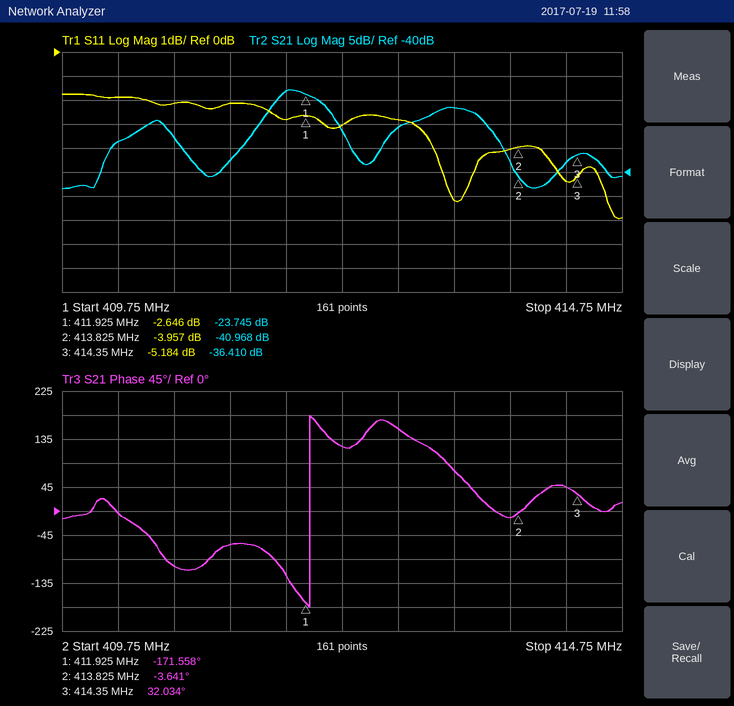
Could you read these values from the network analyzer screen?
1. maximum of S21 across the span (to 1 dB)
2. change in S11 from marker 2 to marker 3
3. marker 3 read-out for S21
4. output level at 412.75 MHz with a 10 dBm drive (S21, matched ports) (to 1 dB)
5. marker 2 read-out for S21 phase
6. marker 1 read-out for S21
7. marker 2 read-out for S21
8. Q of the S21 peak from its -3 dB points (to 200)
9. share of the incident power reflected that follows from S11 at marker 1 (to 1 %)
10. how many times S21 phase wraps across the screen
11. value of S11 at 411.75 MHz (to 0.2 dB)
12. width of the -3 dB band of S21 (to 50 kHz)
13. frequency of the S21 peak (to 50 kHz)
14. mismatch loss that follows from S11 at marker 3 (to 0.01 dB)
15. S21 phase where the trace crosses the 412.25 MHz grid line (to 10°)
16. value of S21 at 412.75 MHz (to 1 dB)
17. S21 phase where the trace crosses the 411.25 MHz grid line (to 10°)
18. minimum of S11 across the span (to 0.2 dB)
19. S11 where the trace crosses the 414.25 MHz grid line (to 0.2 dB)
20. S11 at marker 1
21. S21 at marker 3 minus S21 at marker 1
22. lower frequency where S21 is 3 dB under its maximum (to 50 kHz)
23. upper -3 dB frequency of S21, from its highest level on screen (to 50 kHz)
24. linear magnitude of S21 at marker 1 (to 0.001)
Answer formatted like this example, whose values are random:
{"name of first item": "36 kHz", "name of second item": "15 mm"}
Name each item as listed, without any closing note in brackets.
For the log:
{"maximum of S21 across the span": "-23 dB", "change in S11 from marker 2 to marker 3": "-1.227 dB", "marker 3 read-out for S21": "-36.410 dB", "output level at 412.75 MHz with a 10 dBm drive (S21, matched ports)": "-21 dBm", "marker 2 read-out for S21 phase": "-3.641°", "marker 1 read-out for S21": "-23.745 dB", "marker 2 read-out for S21": "-40.968 dB", "Q of the S21 peak from its -3 dB points": "1000", "share of the incident power reflected that follows from S11 at marker 1": "54 %", "how many times S21 phase wraps across the screen": "1", "value of S11 at 411.75 MHz": "-2.8 dB", "width of the -3 dB band of S21": "450 kHz", "frequency of the S21 peak": "411.80 MHz", "mismatch loss that follows from S11 at marker 3": "1.57 dB", "S21 phase where the trace crosses the 412.25 MHz grid line": "120°", "value of S21 at 412.75 MHz": "-31 dB", "S21 phase where the trace crosses the 411.25 MHz grid line": "-60°", "minimum of S11 across the span": "-7.0 dB", "S11 where the trace crosses the 414.25 MHz grid line": "-5.4 dB", "S11 at marker 1": "-2.646 dB", "S21 at marker 3 minus S21 at marker 1": "-12.665 dB", "lower frequency where S21 is 3 dB under its maximum": "411.65 MHz", "upper -3 dB frequency of S21, from its highest level on screen": "412.10 MHz", "linear magnitude of S21 at marker 1": "0.065"}
